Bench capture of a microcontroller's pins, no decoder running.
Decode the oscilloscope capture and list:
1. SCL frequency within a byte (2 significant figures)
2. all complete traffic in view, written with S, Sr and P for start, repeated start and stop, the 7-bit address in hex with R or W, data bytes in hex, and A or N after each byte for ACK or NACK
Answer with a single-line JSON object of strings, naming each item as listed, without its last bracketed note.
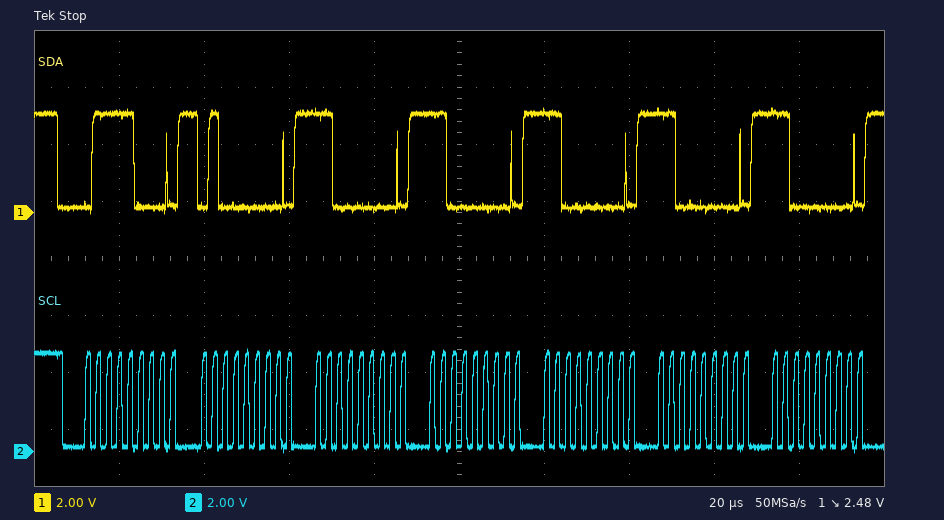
{"SCL frequency within a byte": "400 kHz", "all complete traffic in view, written with S, Sr and P for start, repeated start and stop, the 7-bit address in hex with R or W, data bytes in hex, and A or N after each byte for ACK or NACK": "S 3CW A 40 A C0 A C0 A C0 A C0 A C0 A"}
